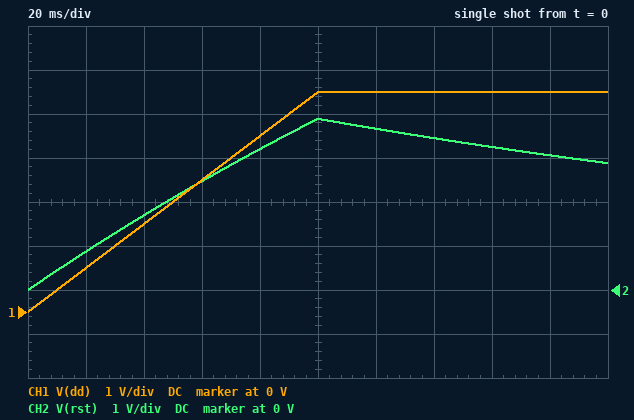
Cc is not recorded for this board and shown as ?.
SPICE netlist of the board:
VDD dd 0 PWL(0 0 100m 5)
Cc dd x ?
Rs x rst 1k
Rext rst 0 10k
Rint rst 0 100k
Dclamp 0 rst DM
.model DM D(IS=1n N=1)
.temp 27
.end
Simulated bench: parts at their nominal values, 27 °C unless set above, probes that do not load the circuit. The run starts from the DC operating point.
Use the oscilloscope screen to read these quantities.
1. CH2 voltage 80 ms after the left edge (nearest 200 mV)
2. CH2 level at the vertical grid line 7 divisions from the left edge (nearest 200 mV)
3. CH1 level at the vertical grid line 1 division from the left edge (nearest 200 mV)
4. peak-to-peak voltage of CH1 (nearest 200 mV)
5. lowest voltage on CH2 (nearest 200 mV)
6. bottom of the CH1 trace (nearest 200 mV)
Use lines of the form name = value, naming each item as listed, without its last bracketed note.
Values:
CH2 voltage 80 ms after the left edge = 3.2 V
CH2 level at the vertical grid line 7 divisions from the left edge = 3.4 V
CH1 level at the vertical grid line 1 division from the left edge = 1.0 V
peak-to-peak voltage of CH1 = 5.0 V
lowest voltage on CH2 = 0 V
bottom of the CH1 trace = 0 V
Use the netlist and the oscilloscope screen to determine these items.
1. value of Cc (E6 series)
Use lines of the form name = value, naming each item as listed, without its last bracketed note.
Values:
value of Cc = 33 µF
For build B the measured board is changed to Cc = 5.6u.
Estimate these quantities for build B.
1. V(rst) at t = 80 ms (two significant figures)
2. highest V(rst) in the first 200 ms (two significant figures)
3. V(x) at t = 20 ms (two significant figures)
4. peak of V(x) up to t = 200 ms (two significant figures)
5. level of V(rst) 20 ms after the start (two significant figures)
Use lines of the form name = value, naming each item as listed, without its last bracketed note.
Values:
V(rst) at t = 80 ms = 1.9 V
highest V(rst) in the first 200 ms = 2.1 V
V(x) at t = 20 ms = 840 mV
peak of V(x) up to t = 200 ms = 2.3 V
level of V(rst) 20 ms after the start = 760 mV
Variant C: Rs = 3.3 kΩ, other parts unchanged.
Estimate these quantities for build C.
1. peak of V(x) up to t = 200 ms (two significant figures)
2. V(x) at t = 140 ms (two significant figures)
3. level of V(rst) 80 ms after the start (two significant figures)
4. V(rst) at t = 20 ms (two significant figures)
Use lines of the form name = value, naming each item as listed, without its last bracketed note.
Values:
peak of V(x) up to t = 200 ms = 4.4 V
V(x) at t = 140 ms = 4.0 V
level of V(rst) 80 ms after the start = 2.7 V
V(rst) at t = 20 ms = 720 mV
